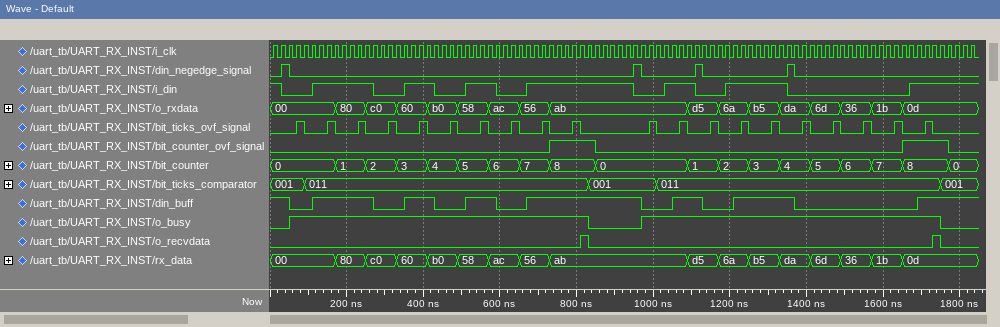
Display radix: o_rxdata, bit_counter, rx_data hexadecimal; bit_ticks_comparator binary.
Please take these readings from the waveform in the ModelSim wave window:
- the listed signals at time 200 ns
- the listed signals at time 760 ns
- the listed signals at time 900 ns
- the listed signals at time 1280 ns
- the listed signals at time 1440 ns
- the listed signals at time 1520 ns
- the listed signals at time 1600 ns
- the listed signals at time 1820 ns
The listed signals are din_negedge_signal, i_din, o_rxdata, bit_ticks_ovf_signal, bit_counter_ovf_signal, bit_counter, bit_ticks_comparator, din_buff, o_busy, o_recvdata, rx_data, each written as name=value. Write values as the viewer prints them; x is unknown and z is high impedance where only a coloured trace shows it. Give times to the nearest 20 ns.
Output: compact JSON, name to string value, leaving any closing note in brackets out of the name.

{"the listed signals at time 200 ns": "din_negedge_signal=0, i_din=1, o_rxdata=80, bit_ticks_ovf_signal=0, bit_counter_ovf_signal=0, bit_counter=1, bit_ticks_comparator=011, din_buff=1, o_busy=1, o_recvdata=0, rx_data=80", "the listed signals at time 760 ns": "din_negedge_signal=0, i_din=1, o_rxdata=ab, bit_ticks_ovf_signal=0, bit_counter_ovf_signal=1, bit_counter=8, bit_ticks_comparator=011, din_buff=1, o_busy=1, o_recvdata=0, rx_data=ab", "the listed signals at time 900 ns": "din_negedge_signal=0, i_din=1, o_rxdata=ab, bit_ticks_ovf_signal=0, bit_counter_ovf_signal=0, bit_counter=0, bit_ticks_comparator=001, din_buff=1, o_busy=0, o_recvdata=0, rx_data=ab", "the listed signals at time 1280 ns": "din_negedge_signal=0, i_din=1, o_rxdata=b5, bit_ticks_ovf_signal=0, bit_counter_ovf_signal=0, bit_counter=3, bit_ticks_comparator=011, din_buff=1, o_busy=1, o_recvdata=0, rx_data=b5", "the listed signals at time 1440 ns": "din_negedge_signal=0, i_din=0, o_rxdata=6d, bit_ticks_ovf_signal=0, bit_counter_ovf_signal=0, bit_counter=5, bit_ticks_comparator=011, din_buff=0, o_busy=1, o_recvdata=0, rx_data=6d", "the listed signals at time 1520 ns": "din_negedge_signal=0, i_din=0, o_rxdata=36, bit_ticks_ovf_signal=0, bit_counter_ovf_signal=0, bit_counter=6, bit_ticks_comparator=011, din_buff=0, o_busy=1, o_recvdata=0, rx_data=36", "the listed signals at time 1600 ns": "din_negedge_signal=0, i_din=0, o_rxdata=1b, bit_ticks_ovf_signal=0, bit_counter_ovf_signal=0, bit_counter=7, bit_ticks_comparator=011, din_buff=0, o_busy=1, o_recvdata=0, rx_data=1b", "the listed signals at time 1820 ns": "din_negedge_signal=0, i_din=1, o_rxdata=0d, bit_ticks_ovf_signal=0, bit_counter_ovf_signal=0, bit_counter=0, bit_ticks_comparator=001, din_buff=1, o_busy=0, o_recvdata=0, rx_data=0d"}
